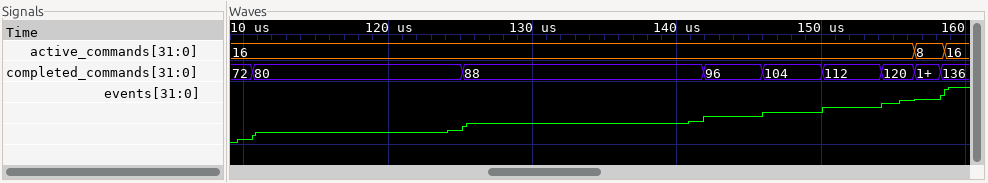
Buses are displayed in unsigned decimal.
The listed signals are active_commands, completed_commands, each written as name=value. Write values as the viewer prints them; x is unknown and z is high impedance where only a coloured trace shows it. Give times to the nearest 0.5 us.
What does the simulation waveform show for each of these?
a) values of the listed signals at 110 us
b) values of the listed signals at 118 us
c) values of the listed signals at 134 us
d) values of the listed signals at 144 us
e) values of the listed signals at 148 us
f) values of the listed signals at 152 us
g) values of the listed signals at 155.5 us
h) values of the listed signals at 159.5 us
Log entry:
active_commands=16, completed_commands=72
active_commands=16, completed_commands=80
active_commands=16, completed_commands=88
active_commands=16, completed_commands=96
active_commands=16, completed_commands=104
active_commands=16, completed_commands=112
active_commands=16, completed_commands=120
active_commands=16, completed_commands=136
